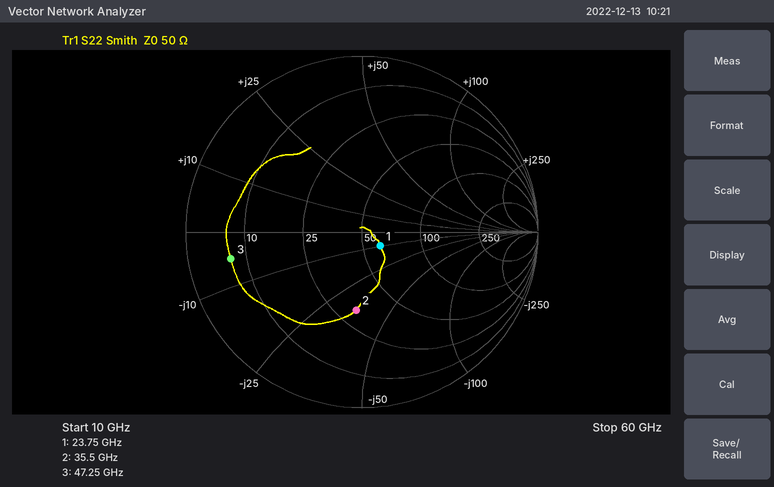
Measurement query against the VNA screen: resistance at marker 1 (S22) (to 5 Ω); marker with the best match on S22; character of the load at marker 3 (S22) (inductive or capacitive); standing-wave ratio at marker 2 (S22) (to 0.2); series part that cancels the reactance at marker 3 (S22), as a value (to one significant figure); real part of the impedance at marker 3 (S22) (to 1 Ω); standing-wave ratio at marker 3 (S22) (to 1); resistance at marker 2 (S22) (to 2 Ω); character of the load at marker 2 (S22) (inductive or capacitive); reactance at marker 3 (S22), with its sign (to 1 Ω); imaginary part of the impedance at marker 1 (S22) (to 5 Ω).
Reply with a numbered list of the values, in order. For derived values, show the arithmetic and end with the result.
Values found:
1. 60 Ω
2. marker 1
3. capacitive
4. 2.6
5. L = 5 Ω/(2π × 47.25 GHz) ≈ 16.8 pH, so 20 pH to one significant figure
6. 7 Ω
7. 7
8. 32 Ω
9. capacitive
10. -5 Ω
11. -10 Ω
